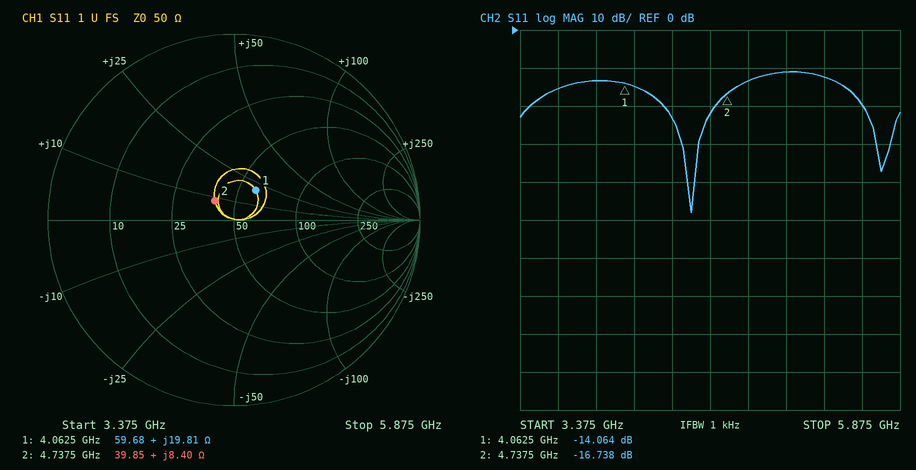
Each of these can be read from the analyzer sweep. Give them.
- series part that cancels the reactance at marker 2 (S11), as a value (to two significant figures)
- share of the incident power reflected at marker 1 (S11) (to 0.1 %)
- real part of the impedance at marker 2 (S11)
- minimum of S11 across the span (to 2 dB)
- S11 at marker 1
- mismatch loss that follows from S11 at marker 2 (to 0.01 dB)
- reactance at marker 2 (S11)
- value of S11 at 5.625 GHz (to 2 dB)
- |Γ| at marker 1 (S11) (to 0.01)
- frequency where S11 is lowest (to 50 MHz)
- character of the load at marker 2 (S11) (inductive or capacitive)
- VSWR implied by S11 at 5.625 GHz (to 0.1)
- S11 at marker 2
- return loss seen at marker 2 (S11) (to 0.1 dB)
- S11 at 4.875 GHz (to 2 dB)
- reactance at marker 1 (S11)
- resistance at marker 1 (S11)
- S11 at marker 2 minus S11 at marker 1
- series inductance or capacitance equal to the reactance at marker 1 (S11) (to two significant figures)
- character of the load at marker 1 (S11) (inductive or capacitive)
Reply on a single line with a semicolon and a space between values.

4.0 pF; 3.9 %; 39.85 Ω; -48 dB; -14.064 dB; 0.09 dB; +8.40 Ω; -20 dB; 0.20; 4.50 GHz; inductive; 1.2; -16.738 dB; 16.7 dB; -14 dB; +19.81 Ω; 59.68 Ω; -2.674 dB; 780 pH; inductive
